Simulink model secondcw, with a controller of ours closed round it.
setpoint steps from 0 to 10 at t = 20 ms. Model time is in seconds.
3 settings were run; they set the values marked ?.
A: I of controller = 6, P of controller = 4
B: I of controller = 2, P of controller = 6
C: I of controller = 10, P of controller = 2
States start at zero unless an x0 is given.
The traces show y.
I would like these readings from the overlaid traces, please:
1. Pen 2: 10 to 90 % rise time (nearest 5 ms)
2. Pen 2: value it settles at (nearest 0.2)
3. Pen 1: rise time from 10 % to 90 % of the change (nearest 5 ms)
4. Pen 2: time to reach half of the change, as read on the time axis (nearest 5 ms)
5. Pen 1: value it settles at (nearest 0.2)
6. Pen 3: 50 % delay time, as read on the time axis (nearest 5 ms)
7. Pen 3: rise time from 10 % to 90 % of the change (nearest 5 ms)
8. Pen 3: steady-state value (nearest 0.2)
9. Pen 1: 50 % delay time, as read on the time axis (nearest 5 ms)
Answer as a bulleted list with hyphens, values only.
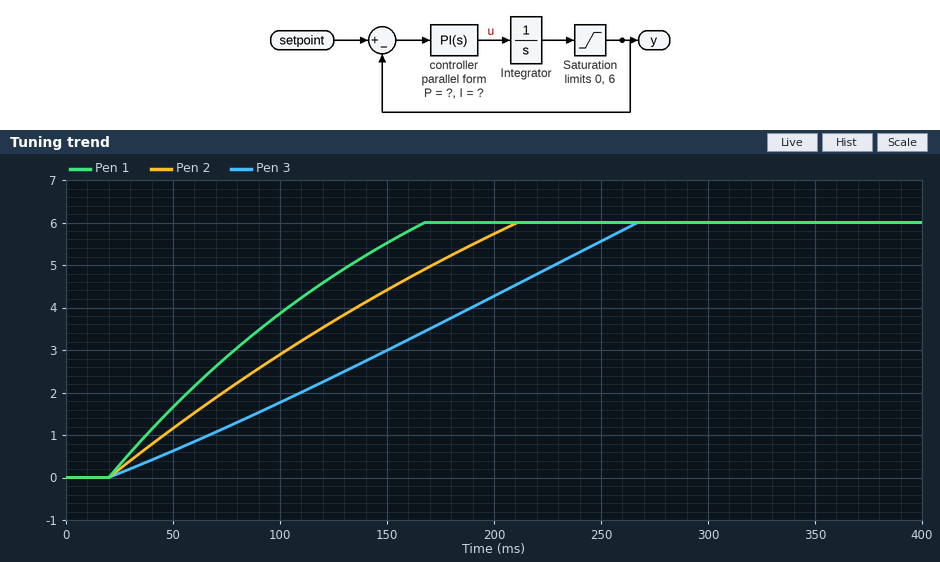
- 150 ms
- 6.0
- 115 ms
- 105 ms
- 6.0
- 150 ms
- 195 ms
- 6.0
- 80 ms
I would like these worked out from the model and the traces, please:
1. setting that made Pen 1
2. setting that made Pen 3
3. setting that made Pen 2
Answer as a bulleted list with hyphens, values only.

- B
- C
- A
